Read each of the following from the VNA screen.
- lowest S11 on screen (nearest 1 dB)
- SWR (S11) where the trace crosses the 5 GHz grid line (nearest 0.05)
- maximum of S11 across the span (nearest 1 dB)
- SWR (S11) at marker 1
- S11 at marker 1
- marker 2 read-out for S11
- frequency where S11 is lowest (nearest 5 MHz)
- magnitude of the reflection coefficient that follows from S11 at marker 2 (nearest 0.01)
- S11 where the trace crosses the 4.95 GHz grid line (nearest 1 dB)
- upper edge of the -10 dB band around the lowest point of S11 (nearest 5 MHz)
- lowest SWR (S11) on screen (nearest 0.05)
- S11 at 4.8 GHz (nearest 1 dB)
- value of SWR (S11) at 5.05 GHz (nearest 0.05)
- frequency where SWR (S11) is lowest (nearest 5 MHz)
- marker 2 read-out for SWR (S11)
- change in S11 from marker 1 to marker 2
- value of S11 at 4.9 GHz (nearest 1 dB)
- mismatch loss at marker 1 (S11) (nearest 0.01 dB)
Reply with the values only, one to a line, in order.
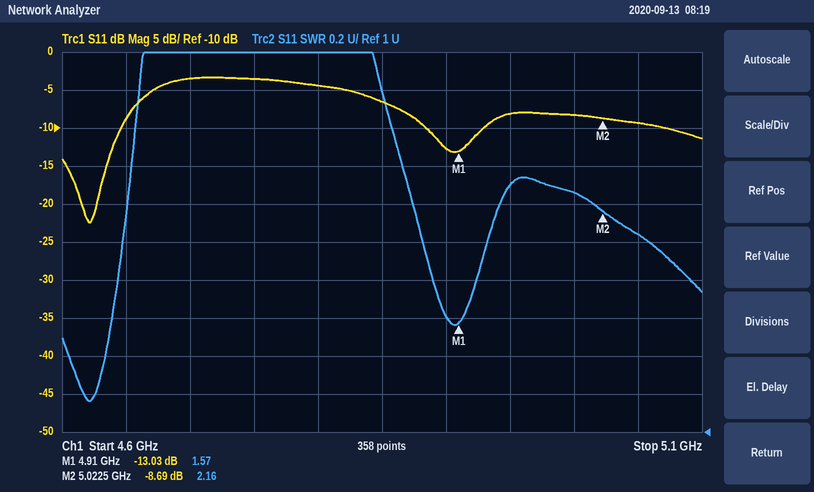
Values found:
-22 dB
2.25
-3 dB
1.57
-13.03 dB
-8.69 dB
4.620 GHz
0.37
-8 dB
4.645 GHz
1.15
-4 dB
2.05
4.620 GHz
2.16
4.34 dB
-13 dB
0.22 dB
